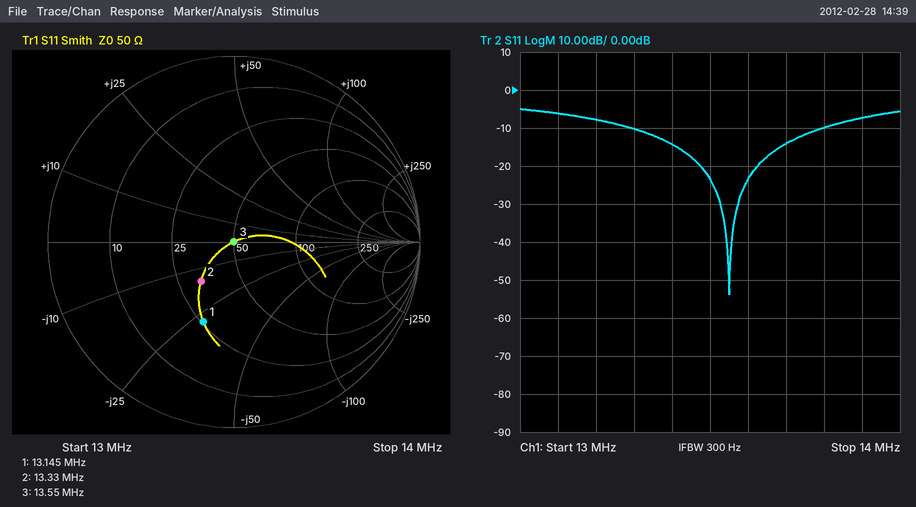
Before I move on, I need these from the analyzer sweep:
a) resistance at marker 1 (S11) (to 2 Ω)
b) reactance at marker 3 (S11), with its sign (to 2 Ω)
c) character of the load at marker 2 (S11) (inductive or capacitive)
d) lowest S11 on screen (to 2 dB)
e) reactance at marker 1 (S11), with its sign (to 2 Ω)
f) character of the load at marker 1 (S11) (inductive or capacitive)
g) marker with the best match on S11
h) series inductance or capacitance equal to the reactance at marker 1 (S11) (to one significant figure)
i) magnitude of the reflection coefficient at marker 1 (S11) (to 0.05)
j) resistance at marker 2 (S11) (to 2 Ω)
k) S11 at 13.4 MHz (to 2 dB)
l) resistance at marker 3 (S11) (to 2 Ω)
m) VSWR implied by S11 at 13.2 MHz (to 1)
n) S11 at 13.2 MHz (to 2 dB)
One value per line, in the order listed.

26 Ω
0 Ω
capacitive
-54 dB
-28 Ω
capacitive
marker 3
400 pF
0.45
32 Ω
-14 dB
50 Ω
2
-8 dB
